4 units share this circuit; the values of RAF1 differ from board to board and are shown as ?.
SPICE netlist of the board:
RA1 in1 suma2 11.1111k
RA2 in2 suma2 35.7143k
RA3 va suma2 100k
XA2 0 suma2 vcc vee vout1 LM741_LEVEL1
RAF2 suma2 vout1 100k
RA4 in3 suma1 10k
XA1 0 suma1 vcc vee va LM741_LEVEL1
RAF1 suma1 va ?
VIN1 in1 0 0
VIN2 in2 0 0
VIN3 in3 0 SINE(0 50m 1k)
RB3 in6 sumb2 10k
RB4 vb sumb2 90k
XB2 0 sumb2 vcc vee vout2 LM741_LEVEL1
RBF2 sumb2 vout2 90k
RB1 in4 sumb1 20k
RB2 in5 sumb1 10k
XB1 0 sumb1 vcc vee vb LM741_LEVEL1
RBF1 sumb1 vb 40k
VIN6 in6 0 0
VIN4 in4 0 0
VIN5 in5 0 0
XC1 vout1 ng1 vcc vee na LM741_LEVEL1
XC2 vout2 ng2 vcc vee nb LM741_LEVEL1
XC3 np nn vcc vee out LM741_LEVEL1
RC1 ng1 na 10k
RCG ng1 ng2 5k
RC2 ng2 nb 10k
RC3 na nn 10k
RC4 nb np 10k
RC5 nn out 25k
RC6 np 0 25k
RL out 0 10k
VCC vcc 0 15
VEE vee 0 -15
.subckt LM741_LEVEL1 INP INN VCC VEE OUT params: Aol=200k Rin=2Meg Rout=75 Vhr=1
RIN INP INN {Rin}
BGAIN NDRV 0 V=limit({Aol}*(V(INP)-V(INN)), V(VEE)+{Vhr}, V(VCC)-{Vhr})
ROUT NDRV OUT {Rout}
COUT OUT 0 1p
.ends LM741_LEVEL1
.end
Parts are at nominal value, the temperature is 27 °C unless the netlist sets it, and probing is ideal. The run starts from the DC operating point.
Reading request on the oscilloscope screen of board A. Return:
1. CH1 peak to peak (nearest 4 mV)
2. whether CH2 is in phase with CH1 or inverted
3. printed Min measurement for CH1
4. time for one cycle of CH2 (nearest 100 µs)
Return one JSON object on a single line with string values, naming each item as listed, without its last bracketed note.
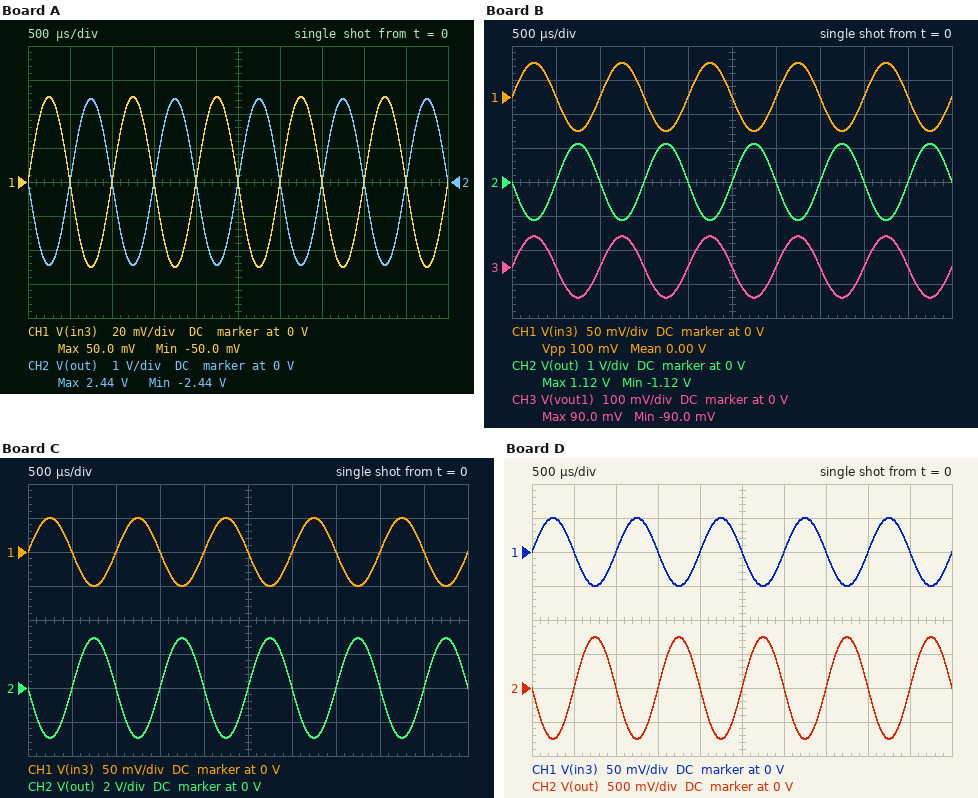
{"CH1 peak to peak": "100 mV", "whether CH2 is in phase with CH1 or inverted": "inverted", "printed Min measurement for CH1": "-50.0 mV", "time for one cycle of CH2": "1.0 ms"}
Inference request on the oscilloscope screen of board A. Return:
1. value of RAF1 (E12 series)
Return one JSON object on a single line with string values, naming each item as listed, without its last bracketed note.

{"value of RAF1": "39 kΩ"}
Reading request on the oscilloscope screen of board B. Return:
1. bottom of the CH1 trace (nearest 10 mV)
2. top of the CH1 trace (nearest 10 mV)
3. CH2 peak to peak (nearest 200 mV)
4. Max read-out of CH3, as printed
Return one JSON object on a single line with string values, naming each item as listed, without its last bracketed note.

{"bottom of the CH1 trace": "-50 mV", "top of the CH1 trace": "50 mV", "CH2 peak to peak": "2.2 V", "Max read-out of CH3, as printed": "90.0 mV"}
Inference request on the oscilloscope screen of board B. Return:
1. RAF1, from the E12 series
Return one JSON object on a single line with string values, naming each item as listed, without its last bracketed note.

{"RAF1, from the E12 series": "18 kΩ"}
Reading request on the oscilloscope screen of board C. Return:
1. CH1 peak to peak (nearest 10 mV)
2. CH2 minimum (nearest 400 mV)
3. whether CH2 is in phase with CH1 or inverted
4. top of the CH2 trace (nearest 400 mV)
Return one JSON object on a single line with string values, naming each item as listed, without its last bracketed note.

{"CH1 peak to peak": "100 mV", "CH2 minimum": "-2.8 V", "whether CH2 is in phase with CH1 or inverted": "inverted", "top of the CH2 trace": "2.8 V"}
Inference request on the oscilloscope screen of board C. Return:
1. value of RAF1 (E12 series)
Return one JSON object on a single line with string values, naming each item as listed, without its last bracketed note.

{"value of RAF1": "47 kΩ"}
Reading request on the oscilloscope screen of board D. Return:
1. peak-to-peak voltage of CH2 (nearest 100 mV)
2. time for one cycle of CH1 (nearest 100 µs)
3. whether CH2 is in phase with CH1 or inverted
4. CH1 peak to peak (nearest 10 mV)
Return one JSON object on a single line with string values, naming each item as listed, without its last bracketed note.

{"peak-to-peak voltage of CH2": "1.5 V", "time for one cycle of CH1": "1.0 ms", "whether CH2 is in phase with CH1 or inverted": "inverted", "CH1 peak to peak": "100 mV"}
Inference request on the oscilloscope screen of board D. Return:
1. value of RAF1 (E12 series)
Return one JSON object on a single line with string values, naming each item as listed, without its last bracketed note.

{"value of RAF1": "12 kΩ"}
